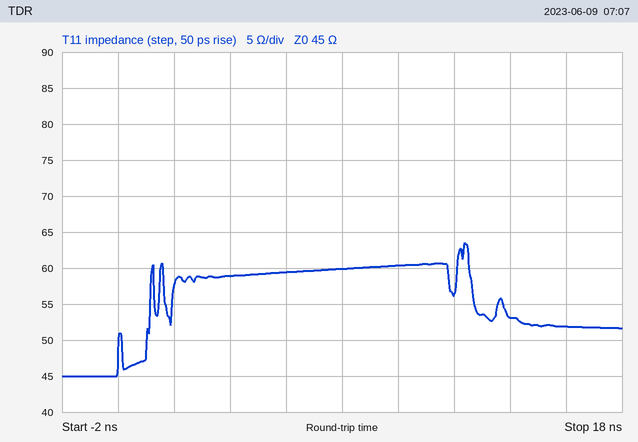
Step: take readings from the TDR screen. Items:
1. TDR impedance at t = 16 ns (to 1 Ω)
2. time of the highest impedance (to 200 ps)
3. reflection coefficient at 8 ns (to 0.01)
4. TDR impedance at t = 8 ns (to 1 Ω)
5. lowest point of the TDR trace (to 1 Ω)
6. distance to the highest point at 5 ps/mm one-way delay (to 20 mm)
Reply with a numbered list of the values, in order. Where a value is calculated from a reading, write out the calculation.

1. 52 Ω
2. 12.4 ns
3. (60 − 45)/(60 + 45) ≈ +0.14
4. 60 Ω
5. 45 Ω
6. 12.4 ns / 2 / 5 ps/mm ≈ 1.24 m
